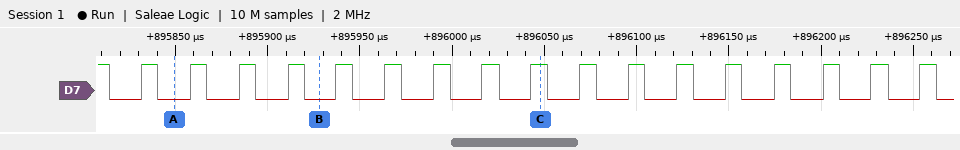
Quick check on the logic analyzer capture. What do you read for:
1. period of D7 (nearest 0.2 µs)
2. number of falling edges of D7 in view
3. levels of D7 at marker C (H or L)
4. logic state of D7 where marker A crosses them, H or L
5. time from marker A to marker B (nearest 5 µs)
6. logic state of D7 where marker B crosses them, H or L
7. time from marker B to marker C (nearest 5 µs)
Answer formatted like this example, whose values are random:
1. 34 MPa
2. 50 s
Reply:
1. 26.4 µs
2. 18
3. D7=H
4. D7=L
5. 80 µs
6. D7=L
7. 120 µs
